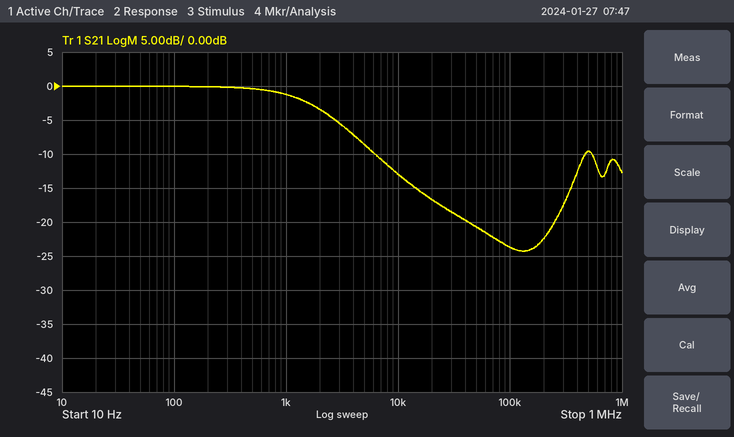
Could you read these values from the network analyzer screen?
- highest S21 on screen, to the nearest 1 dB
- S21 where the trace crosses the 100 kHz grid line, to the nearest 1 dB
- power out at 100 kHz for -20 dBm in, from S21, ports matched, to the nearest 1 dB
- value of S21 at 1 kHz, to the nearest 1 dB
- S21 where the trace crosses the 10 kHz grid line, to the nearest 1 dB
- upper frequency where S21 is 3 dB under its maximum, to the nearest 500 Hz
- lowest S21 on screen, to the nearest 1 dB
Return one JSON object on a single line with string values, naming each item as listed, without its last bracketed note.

{"highest S21 on screen, to the nearest 1 dB": "0 dB", "S21 where the trace crosses the 100 kHz grid line, to the nearest 1 dB": "-24 dB", "power out at 100 kHz for -20 dBm in, from S21, ports matched, to the nearest 1 dB": "-44 dBm", "value of S21 at 1 kHz, to the nearest 1 dB": "-1 dB", "S21 where the trace crosses the 10 kHz grid line, to the nearest 1 dB": "-13 dB", "upper frequency where S21 is 3 dB under its maximum, to the nearest 500 Hz": "2.0 kHz", "lowest S21 on screen, to the nearest 1 dB": "-24 dB"}
